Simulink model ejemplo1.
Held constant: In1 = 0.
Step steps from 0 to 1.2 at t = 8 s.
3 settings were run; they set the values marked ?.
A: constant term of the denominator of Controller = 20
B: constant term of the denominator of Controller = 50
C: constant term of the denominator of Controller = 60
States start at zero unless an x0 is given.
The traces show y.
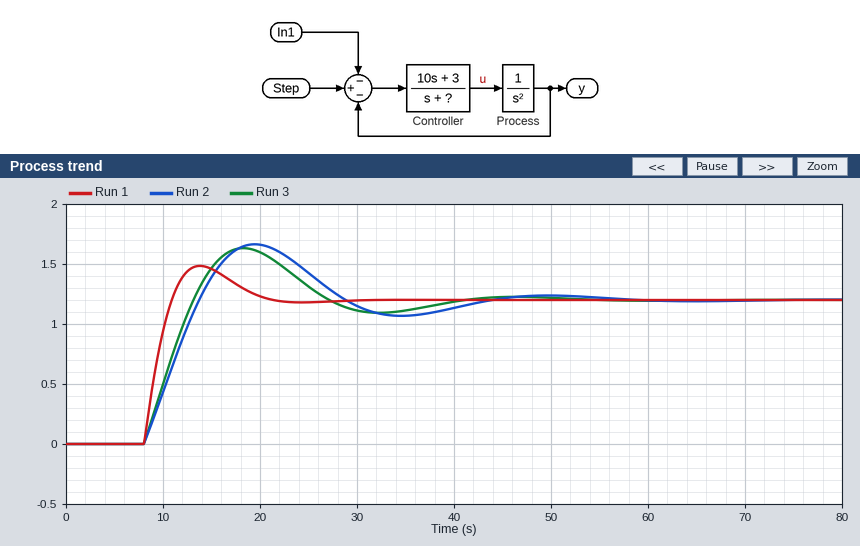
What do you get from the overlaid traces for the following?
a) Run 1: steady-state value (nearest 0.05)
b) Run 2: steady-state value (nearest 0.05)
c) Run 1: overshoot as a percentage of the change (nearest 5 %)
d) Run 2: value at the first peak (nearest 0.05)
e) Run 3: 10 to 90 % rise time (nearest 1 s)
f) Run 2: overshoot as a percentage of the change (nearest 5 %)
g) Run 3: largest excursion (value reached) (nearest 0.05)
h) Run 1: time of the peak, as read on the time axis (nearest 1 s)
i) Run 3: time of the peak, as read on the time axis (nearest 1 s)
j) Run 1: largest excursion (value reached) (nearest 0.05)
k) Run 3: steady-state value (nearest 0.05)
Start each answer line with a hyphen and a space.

- 1.20
- 1.20
- 25 %
- 1.65
- 4 s
- 40 %
- 1.65
- 14 s
- 18 s
- 1.50
- 1.20
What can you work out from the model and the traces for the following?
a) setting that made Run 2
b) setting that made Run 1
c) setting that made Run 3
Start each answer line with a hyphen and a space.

- C
- A
- B
